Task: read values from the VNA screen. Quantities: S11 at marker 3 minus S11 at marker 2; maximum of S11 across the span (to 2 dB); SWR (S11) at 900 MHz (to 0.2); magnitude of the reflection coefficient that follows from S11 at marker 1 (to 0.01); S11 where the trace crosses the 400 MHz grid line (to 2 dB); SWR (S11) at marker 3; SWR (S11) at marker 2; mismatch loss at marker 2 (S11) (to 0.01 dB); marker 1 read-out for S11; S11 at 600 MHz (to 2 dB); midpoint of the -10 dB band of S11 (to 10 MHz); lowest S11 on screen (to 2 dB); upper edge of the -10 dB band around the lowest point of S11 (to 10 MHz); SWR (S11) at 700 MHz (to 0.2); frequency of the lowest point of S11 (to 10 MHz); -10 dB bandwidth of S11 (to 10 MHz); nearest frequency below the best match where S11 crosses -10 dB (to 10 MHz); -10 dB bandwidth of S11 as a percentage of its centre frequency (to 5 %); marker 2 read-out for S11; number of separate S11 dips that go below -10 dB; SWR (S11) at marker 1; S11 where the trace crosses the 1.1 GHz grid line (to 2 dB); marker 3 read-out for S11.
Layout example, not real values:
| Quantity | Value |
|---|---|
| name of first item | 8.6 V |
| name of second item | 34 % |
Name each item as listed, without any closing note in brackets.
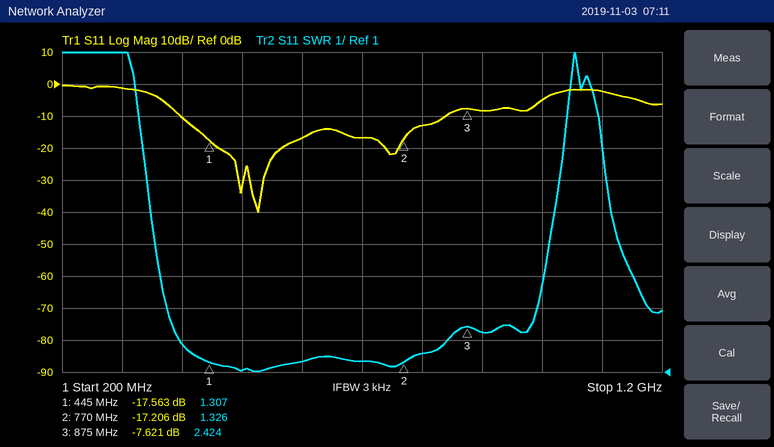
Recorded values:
| Quantity | Value |
|---|---|
| S11 at marker 3 minus S11 at marker 2 | 9.585 dB |
| maximum of S11 across the span | 0 dB |
| SWR (S11) at 900 MHz | 2.2 |
| magnitude of the reflection coefficient that follows from S11 at marker 1 | 0.13 |
| S11 where the trace crosses the 400 MHz grid line | -10 dB |
| SWR (S11) at marker 3 | 2.424 |
| SWR (S11) at marker 2 | 1.326 |
| mismatch loss at marker 2 (S11) | 0.08 dB |
| marker 1 read-out for S11 | -17.563 dB |
| S11 at 600 MHz | -16 dB |
| midpoint of the -10 dB band of S11 | 620 MHz |
| lowest S11 on screen | -40 dB |
| upper edge of the -10 dB band around the lowest point of S11 | 840 MHz |
| SWR (S11) at 700 MHz | 1.4 |
| frequency of the lowest point of S11 | 530 MHz |
| -10 dB bandwidth of S11 | 440 MHz |
| nearest frequency below the best match where S11 crosses -10 dB | 400 MHz |
| -10 dB bandwidth of S11 as a percentage of its centre frequency | 70 % |
| marker 2 read-out for S11 | -17.206 dB |
| number of separate S11 dips that go below -10 dB | 3 |
| SWR (S11) at marker 1 | 1.307 |
| S11 where the trace crosses the 1.1 GHz grid line | -2 dB |
| marker 3 read-out for S11 | -7.621 dB |
